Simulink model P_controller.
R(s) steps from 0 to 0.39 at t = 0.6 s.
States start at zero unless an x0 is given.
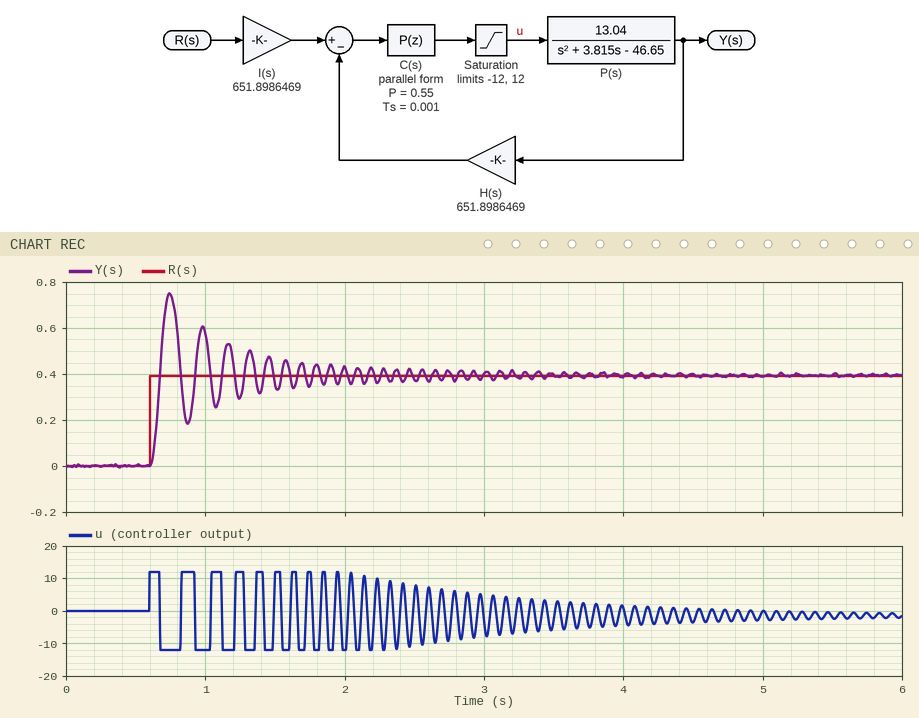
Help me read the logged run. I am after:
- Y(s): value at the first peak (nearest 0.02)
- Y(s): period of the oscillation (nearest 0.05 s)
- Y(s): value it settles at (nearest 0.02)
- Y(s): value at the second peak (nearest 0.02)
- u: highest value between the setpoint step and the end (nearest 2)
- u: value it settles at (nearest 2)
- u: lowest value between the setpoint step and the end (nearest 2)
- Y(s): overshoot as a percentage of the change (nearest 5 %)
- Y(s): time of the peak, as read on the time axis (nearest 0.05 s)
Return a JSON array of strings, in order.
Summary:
["0.74", "0.25 s", "0.40", "0.60", "12", "-2", "-12", "90 %", "0.75 s"]
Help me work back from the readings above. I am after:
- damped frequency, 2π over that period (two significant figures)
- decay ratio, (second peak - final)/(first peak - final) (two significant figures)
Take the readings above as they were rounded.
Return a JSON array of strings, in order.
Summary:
["25 rad/s", "0.59"]
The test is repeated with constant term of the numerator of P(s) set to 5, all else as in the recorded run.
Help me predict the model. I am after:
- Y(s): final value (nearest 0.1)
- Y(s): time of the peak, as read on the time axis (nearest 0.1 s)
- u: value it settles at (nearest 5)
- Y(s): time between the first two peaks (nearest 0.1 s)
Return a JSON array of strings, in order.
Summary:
["0.4", "0.9 s", "-5", "0.4 s"]
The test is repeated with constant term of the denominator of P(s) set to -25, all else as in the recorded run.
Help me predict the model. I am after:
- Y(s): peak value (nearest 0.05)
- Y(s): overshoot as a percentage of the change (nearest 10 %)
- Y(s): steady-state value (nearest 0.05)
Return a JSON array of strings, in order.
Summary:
["0.70", "80 %", "0.40"]
